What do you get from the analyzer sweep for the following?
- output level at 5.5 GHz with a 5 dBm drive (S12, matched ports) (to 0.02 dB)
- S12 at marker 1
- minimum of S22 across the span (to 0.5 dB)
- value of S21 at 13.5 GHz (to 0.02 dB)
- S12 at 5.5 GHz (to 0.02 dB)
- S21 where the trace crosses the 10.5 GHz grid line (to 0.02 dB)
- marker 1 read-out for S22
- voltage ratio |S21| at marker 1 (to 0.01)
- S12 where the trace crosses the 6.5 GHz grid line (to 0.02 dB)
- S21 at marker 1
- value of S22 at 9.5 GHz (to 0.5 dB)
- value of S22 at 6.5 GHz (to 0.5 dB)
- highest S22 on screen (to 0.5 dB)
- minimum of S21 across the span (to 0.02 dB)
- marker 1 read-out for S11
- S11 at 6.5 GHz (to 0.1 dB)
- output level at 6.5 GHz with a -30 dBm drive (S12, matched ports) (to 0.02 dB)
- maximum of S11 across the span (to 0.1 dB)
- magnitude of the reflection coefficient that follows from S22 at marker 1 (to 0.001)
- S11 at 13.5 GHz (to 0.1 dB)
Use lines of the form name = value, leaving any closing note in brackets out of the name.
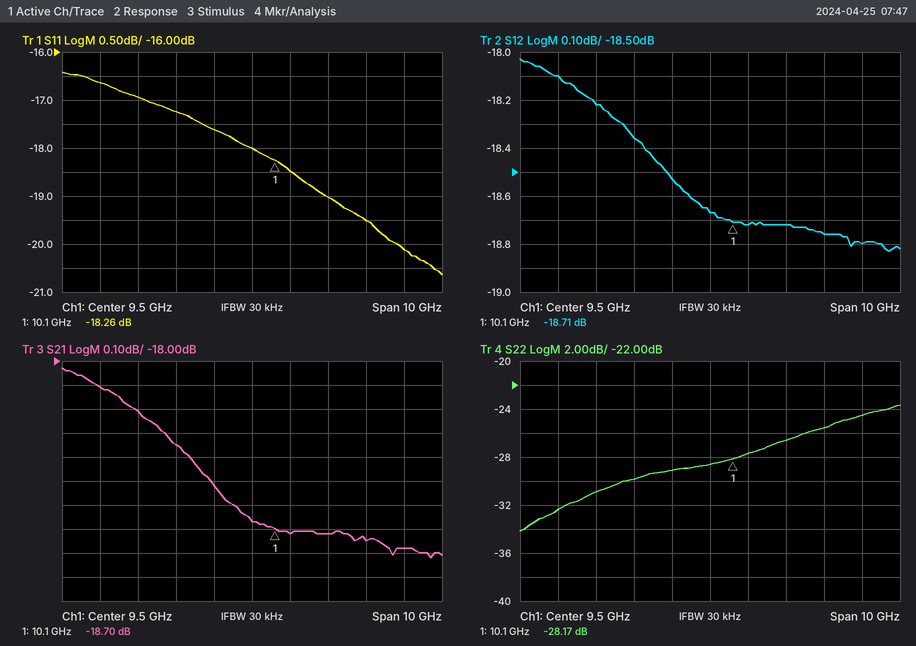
output level at 5.5 GHz with a 5 dBm drive (S12, matched ports) = -13.10 dBm
S12 at marker 1 = -18.71 dB
minimum of S22 across the span = -34.0 dB
value of S21 at 13.5 GHz = -18.78 dB
S12 at 5.5 GHz = -18.10 dB
S21 where the trace crosses the 10.5 GHz grid line = -18.72 dB
marker 1 read-out for S22 = -28.17 dB
voltage ratio |S21| at marker 1 = 0.12
S12 where the trace crosses the 6.5 GHz grid line = -18.22 dB
S21 at marker 1 = -18.70 dB
value of S22 at 9.5 GHz = -28.5 dB
value of S22 at 6.5 GHz = -31.0 dB
highest S22 on screen = -23.5 dB
minimum of S21 across the span = -18.82 dB
marker 1 read-out for S11 = -18.26 dB
S11 at 6.5 GHz = -16.9 dB
output level at 6.5 GHz with a -30 dBm drive (S12, matched ports) = -48.22 dBm
maximum of S11 across the span = -16.4 dB
magnitude of the reflection coefficient that follows from S22 at marker 1 = 0.039
S11 at 13.5 GHz = -20.1 dB
